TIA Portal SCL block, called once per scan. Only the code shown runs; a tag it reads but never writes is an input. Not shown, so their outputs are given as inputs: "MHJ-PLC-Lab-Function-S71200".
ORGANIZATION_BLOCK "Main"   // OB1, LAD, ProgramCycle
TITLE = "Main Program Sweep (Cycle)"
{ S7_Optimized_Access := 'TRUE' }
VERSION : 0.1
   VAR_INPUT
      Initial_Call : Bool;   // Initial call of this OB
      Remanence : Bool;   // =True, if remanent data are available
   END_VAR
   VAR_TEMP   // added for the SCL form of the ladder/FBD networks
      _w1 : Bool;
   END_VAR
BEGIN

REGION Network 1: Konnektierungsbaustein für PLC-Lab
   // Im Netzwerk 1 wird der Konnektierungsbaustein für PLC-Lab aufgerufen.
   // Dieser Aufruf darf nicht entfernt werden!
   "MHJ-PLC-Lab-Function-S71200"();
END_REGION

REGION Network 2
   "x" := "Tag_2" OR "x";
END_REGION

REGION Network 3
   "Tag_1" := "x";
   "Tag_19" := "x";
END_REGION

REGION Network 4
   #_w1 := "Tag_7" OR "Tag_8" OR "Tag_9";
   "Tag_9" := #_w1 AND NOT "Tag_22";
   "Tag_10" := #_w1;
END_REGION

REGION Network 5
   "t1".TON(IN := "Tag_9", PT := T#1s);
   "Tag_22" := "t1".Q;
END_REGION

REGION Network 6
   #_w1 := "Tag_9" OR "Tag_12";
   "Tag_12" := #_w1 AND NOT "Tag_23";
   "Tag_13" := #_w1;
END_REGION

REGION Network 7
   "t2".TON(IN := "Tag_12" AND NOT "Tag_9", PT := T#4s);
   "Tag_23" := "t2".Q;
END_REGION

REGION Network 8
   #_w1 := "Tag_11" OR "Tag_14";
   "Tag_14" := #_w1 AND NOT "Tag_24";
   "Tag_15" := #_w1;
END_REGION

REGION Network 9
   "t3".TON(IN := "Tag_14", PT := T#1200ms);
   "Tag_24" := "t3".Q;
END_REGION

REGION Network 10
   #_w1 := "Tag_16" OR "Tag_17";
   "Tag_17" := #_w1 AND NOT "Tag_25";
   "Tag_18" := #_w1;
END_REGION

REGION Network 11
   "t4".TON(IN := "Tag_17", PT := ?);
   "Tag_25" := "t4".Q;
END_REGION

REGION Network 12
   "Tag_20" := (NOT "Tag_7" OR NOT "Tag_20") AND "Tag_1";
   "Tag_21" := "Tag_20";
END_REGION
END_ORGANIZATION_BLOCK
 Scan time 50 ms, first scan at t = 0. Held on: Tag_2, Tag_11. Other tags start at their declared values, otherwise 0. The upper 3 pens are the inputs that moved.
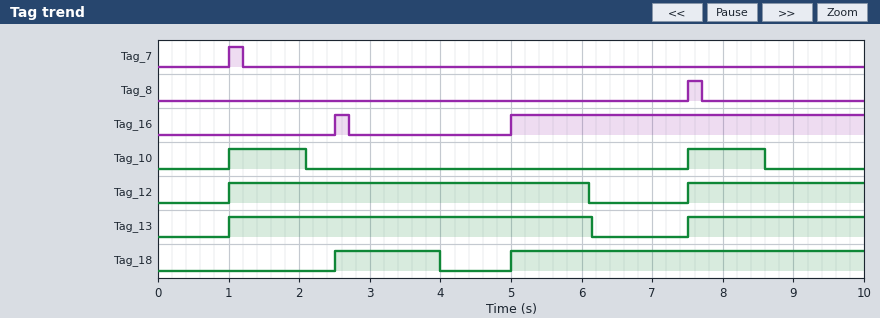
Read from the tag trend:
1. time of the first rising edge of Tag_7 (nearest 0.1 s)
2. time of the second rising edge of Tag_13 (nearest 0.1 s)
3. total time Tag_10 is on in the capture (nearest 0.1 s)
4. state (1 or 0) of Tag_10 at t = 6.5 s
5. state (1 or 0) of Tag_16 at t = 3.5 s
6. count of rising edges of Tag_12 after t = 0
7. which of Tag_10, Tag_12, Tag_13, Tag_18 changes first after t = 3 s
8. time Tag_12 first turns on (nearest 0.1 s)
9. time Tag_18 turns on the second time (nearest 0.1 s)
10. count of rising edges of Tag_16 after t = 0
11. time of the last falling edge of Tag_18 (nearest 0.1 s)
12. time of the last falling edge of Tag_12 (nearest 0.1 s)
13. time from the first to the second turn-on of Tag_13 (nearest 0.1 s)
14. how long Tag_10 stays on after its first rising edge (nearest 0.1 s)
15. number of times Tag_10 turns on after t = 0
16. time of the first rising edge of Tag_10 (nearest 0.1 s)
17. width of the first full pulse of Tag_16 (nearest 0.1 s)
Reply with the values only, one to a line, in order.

1.0 s
7.5 s
2.2 s
0
0
2
Tag_18
1.0 s
5.0 s
2
4.0 s
6.1 s
6.5 s
1.1 s
2
1.0 s
0.2 s
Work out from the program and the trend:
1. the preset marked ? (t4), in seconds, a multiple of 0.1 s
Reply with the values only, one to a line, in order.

1.4 s
